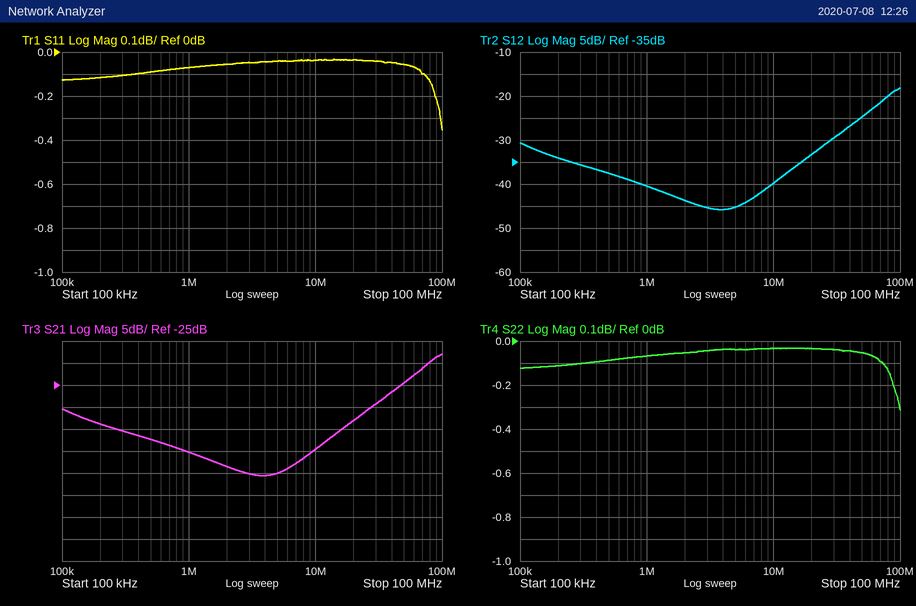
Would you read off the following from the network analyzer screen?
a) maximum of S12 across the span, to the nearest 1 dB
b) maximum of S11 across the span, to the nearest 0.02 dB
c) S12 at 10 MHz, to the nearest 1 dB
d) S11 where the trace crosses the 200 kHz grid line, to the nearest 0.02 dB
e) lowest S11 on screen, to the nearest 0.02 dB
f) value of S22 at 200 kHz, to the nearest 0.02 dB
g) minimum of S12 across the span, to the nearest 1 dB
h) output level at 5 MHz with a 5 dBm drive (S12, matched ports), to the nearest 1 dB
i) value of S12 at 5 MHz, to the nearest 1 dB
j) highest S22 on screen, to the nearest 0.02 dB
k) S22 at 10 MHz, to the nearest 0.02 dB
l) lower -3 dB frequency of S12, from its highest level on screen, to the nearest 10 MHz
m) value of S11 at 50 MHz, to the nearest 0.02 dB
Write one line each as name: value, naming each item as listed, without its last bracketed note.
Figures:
maximum of S12 across the span, to the nearest 1 dB: -18 dB
maximum of S11 across the span, to the nearest 0.02 dB: -0.04 dB
S12 at 10 MHz, to the nearest 1 dB: -40 dB
S11 where the trace crosses the 200 kHz grid line, to the nearest 0.02 dB: -0.12 dB
lowest S11 on screen, to the nearest 0.02 dB: -0.36 dB
value of S22 at 200 kHz, to the nearest 0.02 dB: -0.12 dB
minimum of S12 across the span, to the nearest 1 dB: -46 dB
output level at 5 MHz with a 5 dBm drive (S12, matched ports), to the nearest 1 dB: -40 dBm
value of S12 at 5 MHz, to the nearest 1 dB: -45 dB
highest S22 on screen, to the nearest 0.02 dB: -0.04 dB
S22 at 10 MHz, to the nearest 0.02 dB: -0.04 dB
lower -3 dB frequency of S12, from its highest level on screen, to the nearest 10 MHz: 70 MHz
value of S11 at 50 MHz, to the nearest 0.02 dB: -0.06 dB
